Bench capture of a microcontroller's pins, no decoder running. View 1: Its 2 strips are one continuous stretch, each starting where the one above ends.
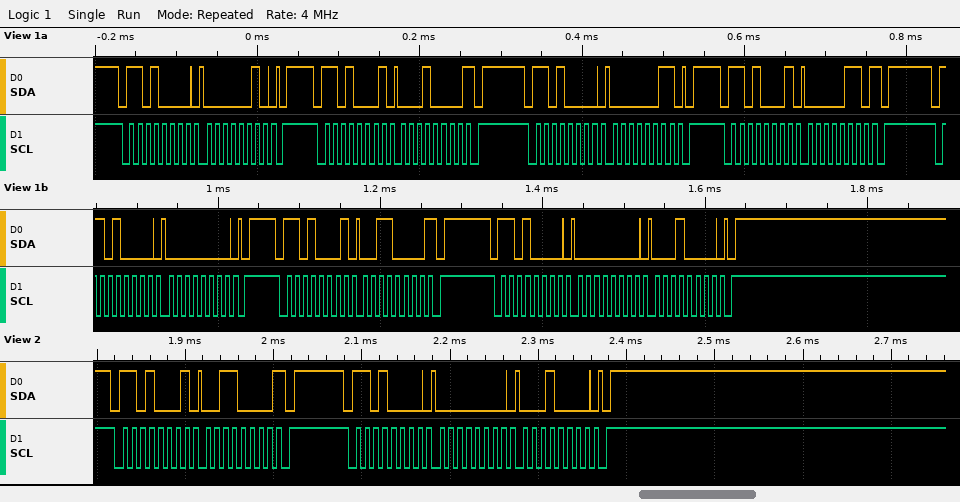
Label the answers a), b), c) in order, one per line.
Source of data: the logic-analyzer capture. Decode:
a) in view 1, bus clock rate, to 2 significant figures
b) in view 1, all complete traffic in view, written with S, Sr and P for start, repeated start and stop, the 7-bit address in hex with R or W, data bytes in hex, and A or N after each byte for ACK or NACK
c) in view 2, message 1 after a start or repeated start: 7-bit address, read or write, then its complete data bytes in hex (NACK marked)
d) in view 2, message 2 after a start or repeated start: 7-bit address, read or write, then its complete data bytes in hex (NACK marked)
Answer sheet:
a) 100 kHz
b) S 68W A 02 A P S 68R A 10 N P S 68W A 03 A P S 68R A 06 N P S 68W A 00 A P S 68R A 30 N P S 68W A 00 A 10 A P
c) 0x68 read: 30 NACK
d) 0x68 write: 00 10
